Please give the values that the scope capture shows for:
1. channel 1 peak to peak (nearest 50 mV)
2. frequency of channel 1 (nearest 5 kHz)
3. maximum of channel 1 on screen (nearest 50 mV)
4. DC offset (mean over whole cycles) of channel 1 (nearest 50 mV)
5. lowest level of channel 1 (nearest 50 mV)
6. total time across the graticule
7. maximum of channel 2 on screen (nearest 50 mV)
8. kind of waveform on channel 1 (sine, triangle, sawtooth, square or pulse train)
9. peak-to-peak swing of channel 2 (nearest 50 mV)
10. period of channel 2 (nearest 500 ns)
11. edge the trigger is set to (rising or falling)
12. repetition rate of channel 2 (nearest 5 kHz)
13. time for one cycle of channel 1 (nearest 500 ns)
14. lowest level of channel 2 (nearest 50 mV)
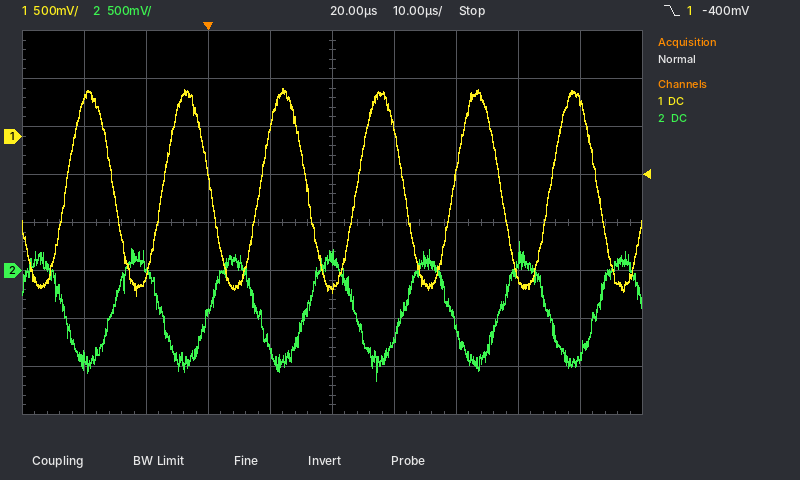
2.15 V
65 kHz
500 mV
-550 mV
-1.65 V
100 µs
300 mV
sine
1.45 V
15.5 µs
falling
65 kHz
15.5 µs
-1.15 V
